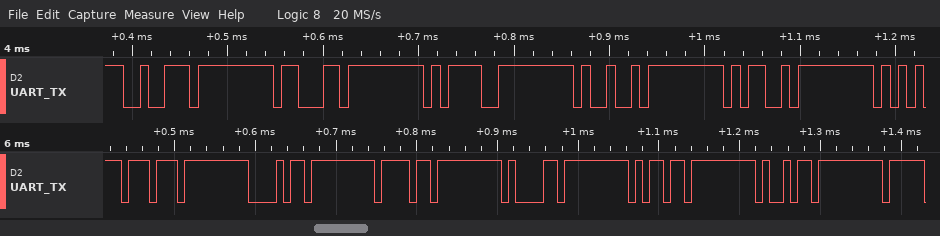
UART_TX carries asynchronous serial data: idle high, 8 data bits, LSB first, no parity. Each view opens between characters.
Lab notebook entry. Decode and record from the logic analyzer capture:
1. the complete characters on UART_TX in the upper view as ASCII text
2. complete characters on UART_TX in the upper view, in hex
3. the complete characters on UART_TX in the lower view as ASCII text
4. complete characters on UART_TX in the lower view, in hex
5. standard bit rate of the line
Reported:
"rc=IM"
72, 63, 3D, 49, 4D
"whoami"
77, 68, 6F, 61, 6D, 69
115200 baud
